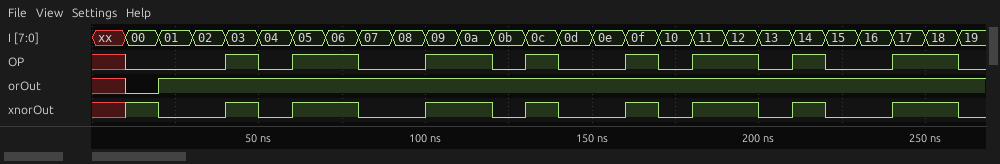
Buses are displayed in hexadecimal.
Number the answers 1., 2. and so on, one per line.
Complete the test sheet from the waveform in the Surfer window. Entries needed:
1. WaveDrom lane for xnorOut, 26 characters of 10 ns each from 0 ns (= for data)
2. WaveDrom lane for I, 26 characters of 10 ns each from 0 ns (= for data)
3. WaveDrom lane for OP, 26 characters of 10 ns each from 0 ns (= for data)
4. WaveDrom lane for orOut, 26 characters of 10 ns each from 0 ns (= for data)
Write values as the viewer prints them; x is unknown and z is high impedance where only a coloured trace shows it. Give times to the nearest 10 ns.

1. {name: 'xnorOut', wave: 'x10.101.0.1.010.101.010.1.'}
2. {name: 'I', wave: 'x=========================', data: '00 01 02 03 04 05 06 07 08 09 0a 0b 0c 0d 0e 0f 10 11 12 13 14 15 16 17 18'}
3. {name: 'OP', wave: 'x0..101.0.1.010.101.010.1.'}
4. {name: 'orOut', wave: 'x01.......................'}
